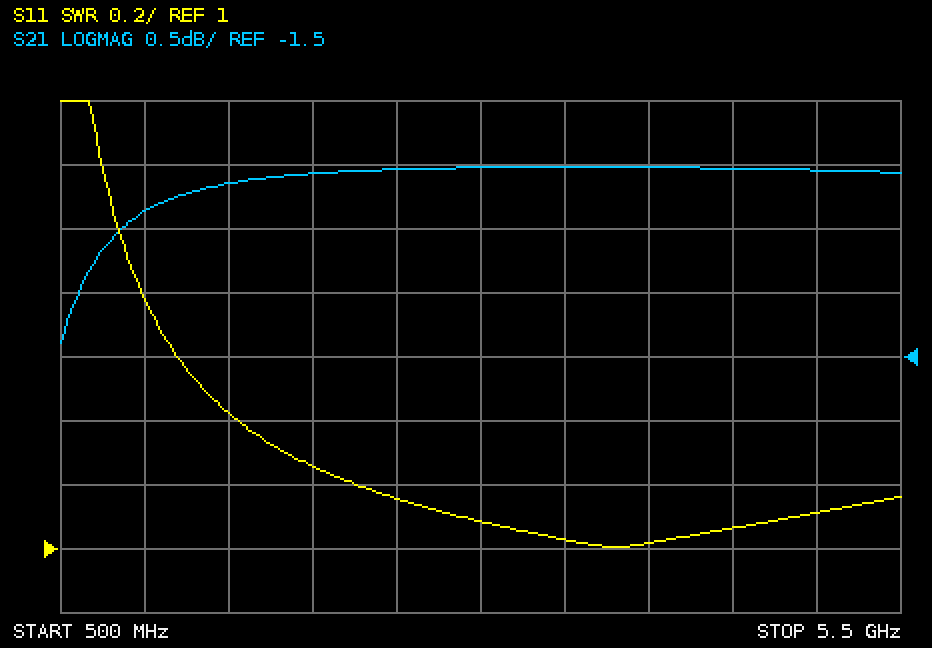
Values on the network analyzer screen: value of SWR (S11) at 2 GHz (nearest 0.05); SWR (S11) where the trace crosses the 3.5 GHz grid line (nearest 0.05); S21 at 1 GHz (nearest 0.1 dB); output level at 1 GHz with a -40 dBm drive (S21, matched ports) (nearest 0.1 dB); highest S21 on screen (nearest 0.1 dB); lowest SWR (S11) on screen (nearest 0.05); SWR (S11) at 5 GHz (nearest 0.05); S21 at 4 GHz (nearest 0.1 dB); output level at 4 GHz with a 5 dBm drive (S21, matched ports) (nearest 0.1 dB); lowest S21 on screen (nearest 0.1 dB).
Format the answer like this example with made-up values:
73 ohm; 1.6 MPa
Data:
1.25; 1.05; -0.4 dB; -40.4 dBm; 0.0 dB; 1.00; 1.10; 0.0 dB; 5.0 dBm; -1.4 dB
